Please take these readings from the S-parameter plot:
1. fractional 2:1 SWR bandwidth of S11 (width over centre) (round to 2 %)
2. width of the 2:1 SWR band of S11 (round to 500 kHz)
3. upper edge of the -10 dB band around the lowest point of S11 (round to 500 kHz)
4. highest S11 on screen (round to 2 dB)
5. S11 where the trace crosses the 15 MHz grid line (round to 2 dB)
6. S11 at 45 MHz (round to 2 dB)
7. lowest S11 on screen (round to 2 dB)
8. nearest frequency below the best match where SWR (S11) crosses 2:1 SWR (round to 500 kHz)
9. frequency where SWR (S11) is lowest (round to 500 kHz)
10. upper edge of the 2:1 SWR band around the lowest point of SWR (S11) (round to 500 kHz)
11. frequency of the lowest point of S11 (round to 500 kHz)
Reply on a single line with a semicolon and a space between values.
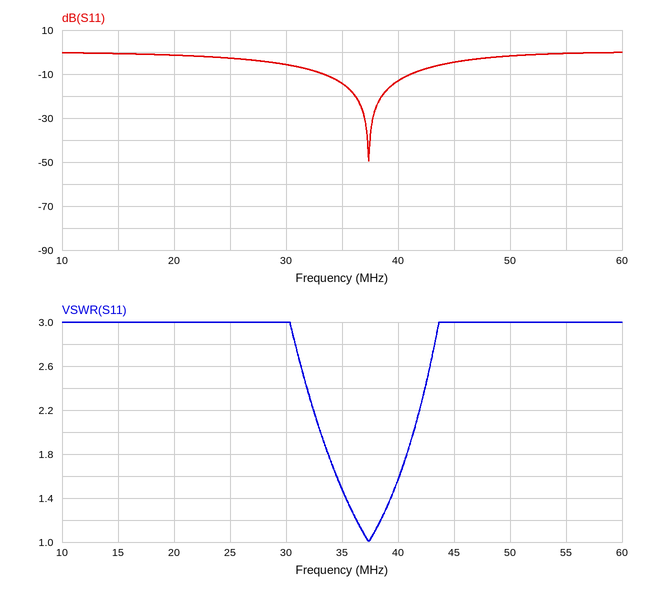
22 %; 8.5 MHz; 41.0 MHz; 0 dB; 0 dB; -4 dB; -50 dB; 33.0 MHz; 37.5 MHz; 41.5 MHz; 37.5 MHz
